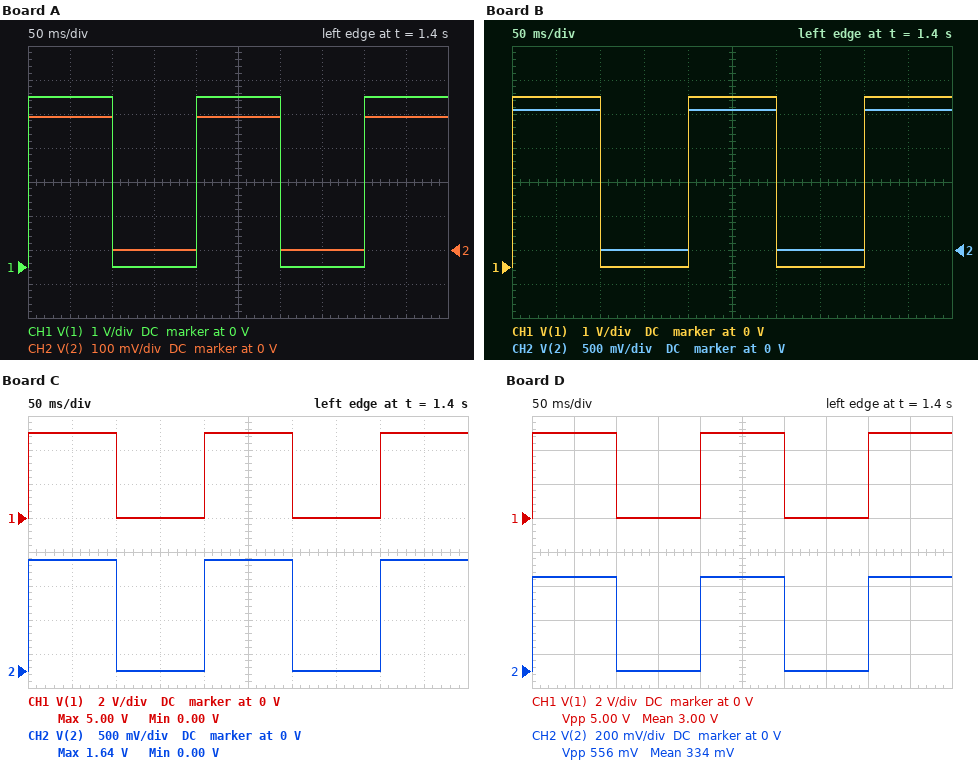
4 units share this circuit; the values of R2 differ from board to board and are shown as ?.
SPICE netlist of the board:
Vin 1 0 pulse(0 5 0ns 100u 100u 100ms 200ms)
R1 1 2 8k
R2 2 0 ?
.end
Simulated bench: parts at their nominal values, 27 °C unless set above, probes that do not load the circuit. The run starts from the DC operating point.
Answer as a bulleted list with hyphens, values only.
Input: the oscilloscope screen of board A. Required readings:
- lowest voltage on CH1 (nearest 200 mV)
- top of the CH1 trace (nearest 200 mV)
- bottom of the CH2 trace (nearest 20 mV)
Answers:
- 0 V
- 5.0 V
- 0 V
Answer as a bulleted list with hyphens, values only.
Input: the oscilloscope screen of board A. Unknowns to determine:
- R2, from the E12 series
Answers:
- 680 Ω
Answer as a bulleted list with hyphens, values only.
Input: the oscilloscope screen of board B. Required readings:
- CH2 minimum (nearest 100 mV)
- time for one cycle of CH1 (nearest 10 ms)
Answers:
- 0 V
- 200 ms
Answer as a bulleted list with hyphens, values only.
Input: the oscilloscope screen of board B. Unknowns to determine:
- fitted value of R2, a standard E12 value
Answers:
- 5.6 kΩ
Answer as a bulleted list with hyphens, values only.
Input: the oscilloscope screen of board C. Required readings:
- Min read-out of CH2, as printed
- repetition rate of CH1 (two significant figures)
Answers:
- 0.00 V
- 5.0 Hz
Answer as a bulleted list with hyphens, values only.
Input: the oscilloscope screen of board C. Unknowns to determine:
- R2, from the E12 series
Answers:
- 3.9 kΩ
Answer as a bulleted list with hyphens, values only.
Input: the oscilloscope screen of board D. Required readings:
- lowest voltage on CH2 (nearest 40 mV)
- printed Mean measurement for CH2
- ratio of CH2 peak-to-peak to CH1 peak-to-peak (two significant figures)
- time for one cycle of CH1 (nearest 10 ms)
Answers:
- 0 V
- 334 mV
- 0.11
- 200 ms
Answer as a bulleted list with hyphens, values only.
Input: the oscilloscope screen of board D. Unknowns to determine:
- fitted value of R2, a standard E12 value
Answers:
- 1 kΩ
